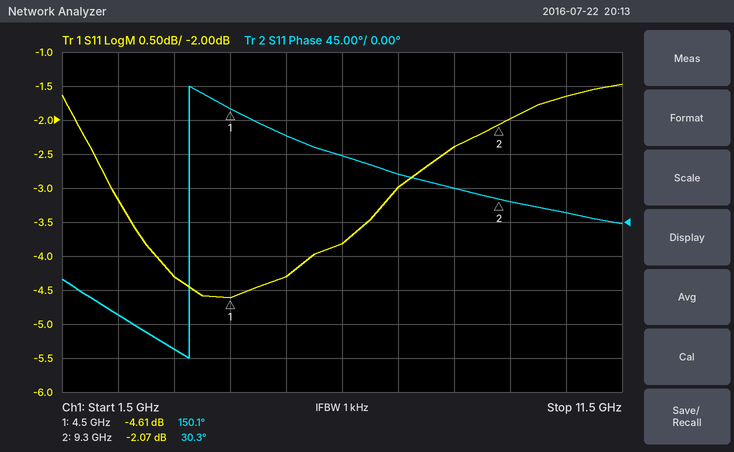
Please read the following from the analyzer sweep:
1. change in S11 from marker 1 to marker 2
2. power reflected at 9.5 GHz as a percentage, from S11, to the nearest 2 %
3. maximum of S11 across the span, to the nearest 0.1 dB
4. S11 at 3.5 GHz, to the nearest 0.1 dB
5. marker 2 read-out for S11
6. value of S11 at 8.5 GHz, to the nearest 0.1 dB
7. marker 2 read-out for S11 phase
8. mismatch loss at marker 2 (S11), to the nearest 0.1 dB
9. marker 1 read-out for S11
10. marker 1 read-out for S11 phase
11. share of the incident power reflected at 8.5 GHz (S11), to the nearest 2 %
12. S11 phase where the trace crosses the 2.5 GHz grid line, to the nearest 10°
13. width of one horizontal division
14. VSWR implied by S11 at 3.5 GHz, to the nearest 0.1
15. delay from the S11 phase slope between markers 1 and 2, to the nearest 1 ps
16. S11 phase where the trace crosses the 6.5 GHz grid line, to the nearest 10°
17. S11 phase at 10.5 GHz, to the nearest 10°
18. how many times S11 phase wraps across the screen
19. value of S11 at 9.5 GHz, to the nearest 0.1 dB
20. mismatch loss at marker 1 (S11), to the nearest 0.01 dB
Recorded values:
2.54 dB
64 %
-1.5 dB
-4.3 dB
-2.07 dB
-2.4 dB
30.3°
4.2 dB
-4.61 dB
150.1°
58 %
-120°
1 GHz
4.1
69 ps
90°
10°
1
-2.0 dB
1.84 dB
